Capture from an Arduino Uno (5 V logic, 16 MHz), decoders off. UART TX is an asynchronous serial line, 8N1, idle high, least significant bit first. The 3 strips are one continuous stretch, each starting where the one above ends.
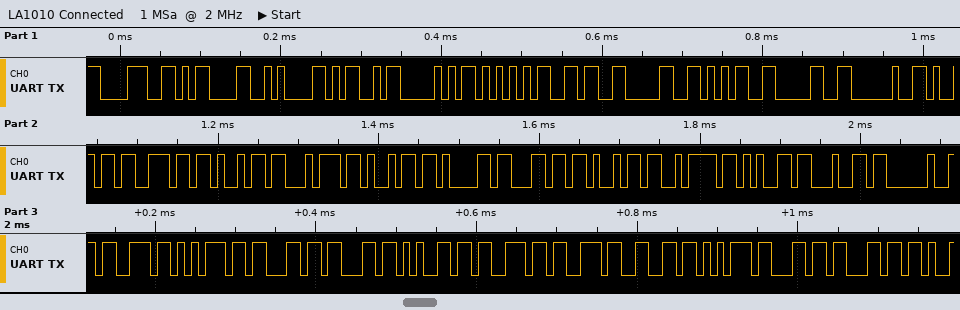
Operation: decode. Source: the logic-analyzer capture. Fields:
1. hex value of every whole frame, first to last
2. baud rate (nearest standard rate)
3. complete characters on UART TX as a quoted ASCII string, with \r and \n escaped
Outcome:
0x38 0x0D 0x0A 0x4D 0x50 0x55 0x36 0x30 0x35 0x30 0x20 0x69 0x6E 0x69 0x74 0x69 0x61 0x6C 0x69 0x7A 0x65 0x64 0x20 0x73 0x75 0x63 0x63 0x65 0x73 0x73 0x66 0x75 0x6C 0x6C
115200 baud
"8\r\nMPU6050 initialized successfull"
